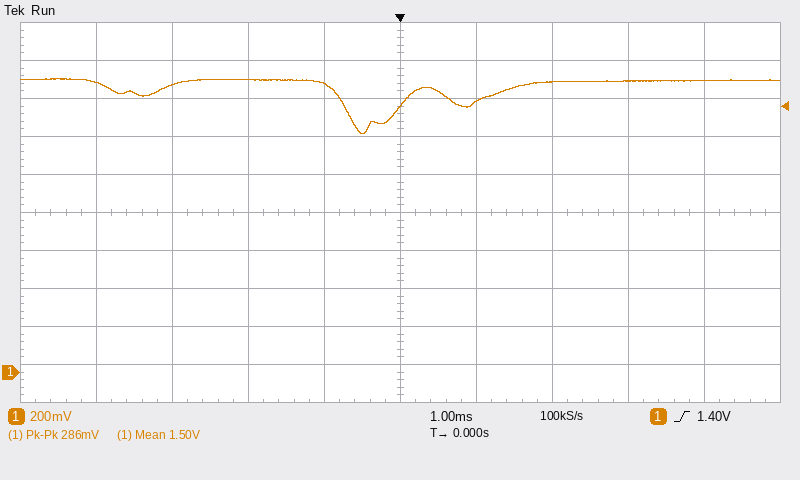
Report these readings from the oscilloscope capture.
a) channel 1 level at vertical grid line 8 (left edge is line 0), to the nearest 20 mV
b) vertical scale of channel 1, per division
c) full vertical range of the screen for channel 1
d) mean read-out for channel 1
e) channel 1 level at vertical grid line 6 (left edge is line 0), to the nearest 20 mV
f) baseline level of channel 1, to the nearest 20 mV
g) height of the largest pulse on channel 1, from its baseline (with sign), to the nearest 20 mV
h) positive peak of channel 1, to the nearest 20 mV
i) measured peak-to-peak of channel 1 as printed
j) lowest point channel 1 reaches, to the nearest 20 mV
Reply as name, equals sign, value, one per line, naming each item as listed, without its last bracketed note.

channel 1 level at vertical grid line 8 (left edge is line 0), to the nearest 20 mV = 1.54 V
vertical scale of channel 1, per division = 200 mV
full vertical range of the screen for channel 1 = 2 V
mean read-out for channel 1 = 1.50 V
channel 1 level at vertical grid line 6 (left edge is line 0), to the nearest 20 mV = 1.42 V
baseline level of channel 1, to the nearest 20 mV = 1.54 V
height of the largest pulse on channel 1, from its baseline (with sign), to the nearest 20 mV = -280 mV
positive peak of channel 1, to the nearest 20 mV = 1.54 V
measured peak-to-peak of channel 1 as printed = 286 mV
lowest point channel 1 reaches, to the nearest 20 mV = 1.26 V
